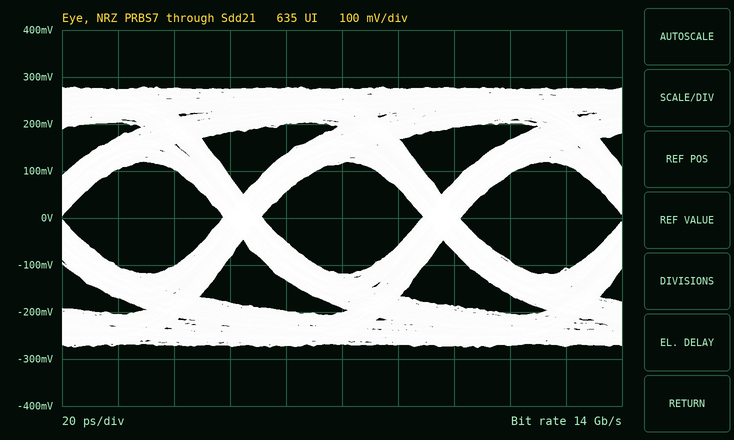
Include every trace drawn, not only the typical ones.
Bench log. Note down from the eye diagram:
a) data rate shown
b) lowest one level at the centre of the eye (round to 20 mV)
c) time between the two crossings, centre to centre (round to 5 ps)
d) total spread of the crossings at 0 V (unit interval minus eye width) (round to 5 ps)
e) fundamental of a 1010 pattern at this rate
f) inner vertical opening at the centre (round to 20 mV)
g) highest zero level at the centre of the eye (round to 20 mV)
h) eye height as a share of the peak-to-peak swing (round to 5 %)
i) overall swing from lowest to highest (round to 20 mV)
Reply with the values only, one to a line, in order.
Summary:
14 Gb/s
120 mV
70 ps
15 ps
7 GHz
240 mV
-120 mV
45 %
560 mV
